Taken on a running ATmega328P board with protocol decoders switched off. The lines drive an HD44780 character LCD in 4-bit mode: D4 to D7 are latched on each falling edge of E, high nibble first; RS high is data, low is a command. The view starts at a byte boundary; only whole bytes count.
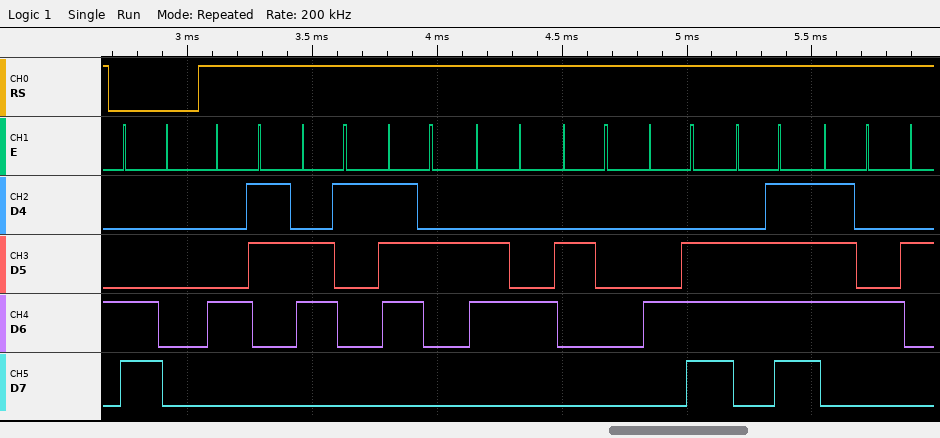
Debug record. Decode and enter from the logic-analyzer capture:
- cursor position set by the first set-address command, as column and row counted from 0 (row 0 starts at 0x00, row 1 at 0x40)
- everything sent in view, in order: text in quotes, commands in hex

column 0, row 1
0xC0 "Card Not"
